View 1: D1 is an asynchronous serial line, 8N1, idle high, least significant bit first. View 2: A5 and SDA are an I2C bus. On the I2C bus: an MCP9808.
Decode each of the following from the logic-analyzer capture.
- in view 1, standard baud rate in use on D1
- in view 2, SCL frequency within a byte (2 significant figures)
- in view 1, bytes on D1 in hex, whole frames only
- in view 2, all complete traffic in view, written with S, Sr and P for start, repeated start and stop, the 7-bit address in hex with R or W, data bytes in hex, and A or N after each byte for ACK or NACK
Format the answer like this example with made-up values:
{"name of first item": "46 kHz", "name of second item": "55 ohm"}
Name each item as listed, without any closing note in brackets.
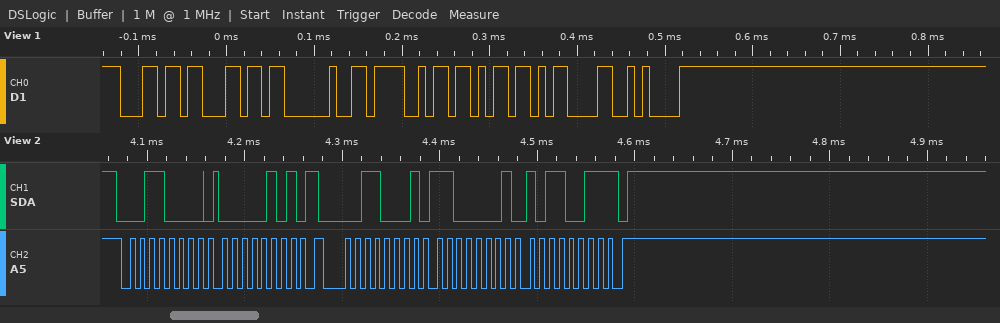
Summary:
{"in view 1, standard baud rate in use on D1": "115200 baud", "in view 2, SCL frequency within a byte": "100 kHz", "in view 1, bytes on D1 in hex, whole frames only": "6C 6C 20 4F 6B 0D 0A", "in view 2, all complete traffic in view, written with S, Sr and P for start, repeated start and stop, the 7-bit address in hex with R or W, data bytes in hex, and A or N after each byte for ACK or NACK": "S 18W A 05 A Sr 18R A C1 A B3 N P"}
